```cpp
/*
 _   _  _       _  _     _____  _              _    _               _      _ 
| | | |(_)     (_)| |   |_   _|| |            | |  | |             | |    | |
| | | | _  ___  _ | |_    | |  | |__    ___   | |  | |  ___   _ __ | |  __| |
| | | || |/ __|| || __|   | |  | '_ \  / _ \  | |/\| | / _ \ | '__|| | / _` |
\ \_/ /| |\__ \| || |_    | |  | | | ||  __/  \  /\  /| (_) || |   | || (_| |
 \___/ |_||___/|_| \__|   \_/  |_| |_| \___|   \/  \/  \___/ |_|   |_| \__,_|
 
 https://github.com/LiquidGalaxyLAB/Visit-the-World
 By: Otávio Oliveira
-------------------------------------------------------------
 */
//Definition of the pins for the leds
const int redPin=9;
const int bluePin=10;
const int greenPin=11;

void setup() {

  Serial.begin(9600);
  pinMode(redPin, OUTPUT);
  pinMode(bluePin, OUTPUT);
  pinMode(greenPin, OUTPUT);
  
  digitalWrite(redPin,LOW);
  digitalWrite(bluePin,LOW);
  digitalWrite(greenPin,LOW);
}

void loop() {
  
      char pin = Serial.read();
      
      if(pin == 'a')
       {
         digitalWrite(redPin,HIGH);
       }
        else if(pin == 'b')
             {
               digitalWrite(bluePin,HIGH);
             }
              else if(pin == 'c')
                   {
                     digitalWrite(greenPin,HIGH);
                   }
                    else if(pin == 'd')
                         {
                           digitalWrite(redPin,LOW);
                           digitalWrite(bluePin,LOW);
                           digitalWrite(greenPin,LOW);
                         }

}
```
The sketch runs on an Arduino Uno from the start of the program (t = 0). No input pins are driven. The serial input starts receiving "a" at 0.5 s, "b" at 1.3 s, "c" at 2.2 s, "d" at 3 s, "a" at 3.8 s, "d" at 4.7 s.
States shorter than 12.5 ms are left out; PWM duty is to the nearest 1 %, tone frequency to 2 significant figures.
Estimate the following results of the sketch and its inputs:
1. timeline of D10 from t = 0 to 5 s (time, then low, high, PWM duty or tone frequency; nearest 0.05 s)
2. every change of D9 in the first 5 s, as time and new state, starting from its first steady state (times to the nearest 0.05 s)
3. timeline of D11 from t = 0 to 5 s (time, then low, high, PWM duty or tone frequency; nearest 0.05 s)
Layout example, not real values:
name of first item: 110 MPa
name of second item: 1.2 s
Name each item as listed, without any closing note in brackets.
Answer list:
timeline of D10 from t = 0 to 5 s: 0 s low; 1.3 s high; 3 s low
every change of D9 in the first 5 s, as time and new state, starting from its first steady state: 0 s low; 0.5 s high; 3 s low; 3.8 s high; 4.7 s low
timeline of D11 from t = 0 to 5 s: 0 s low; 2.2 s high; 3 s low
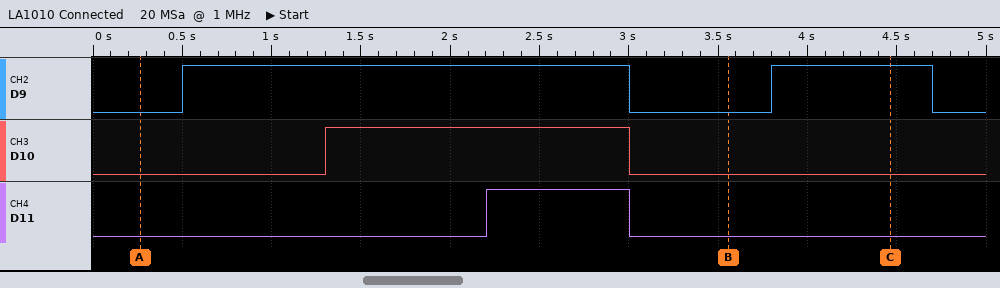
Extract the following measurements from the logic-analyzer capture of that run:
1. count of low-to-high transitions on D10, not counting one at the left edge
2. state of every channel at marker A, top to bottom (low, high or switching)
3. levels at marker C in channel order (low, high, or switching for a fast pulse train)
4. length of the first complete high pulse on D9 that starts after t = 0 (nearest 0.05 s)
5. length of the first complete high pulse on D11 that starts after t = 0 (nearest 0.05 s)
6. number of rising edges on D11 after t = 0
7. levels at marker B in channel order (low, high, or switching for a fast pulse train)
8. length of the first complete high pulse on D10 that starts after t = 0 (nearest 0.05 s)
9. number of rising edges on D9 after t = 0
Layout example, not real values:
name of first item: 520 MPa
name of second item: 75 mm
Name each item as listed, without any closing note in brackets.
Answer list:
count of low-to-high transitions on D10, not counting one at the left edge: 1
state of every channel at marker A, top to bottom: D9 low, D10 low, D11 low
levels at marker C in channel order: D9 high, D10 low, D11 low
length of the first complete high pulse on D9 that starts after t = 0: 2.50 s
length of the first complete high pulse on D11 that starts after t = 0: 0.80 s
number of rising edges on D11 after t = 0: 1
levels at marker B in channel order: D9 low, D10 low, D11 low
length of the first complete high pulse on D10 that starts after t = 0: 1.70 s
number of rising edges on D9 after t = 0: 2
